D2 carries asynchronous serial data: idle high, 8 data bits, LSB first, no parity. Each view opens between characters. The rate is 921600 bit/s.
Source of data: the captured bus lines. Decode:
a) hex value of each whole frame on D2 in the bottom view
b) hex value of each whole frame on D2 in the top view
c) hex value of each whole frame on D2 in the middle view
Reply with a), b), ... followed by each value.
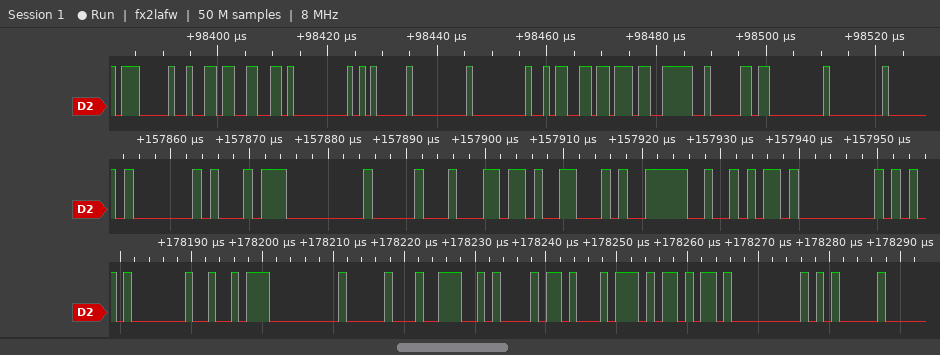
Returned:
a) 01, D2, 00, 10, 4E, 68, 74, 6B, 00, 05
b) 07, B2, 66, 00, 05, 00, 00, 9A, BB, 3E, B0, 00, 00
c) 01, D1, 00, 10, 6C, 46, 3E, 6A, 00
